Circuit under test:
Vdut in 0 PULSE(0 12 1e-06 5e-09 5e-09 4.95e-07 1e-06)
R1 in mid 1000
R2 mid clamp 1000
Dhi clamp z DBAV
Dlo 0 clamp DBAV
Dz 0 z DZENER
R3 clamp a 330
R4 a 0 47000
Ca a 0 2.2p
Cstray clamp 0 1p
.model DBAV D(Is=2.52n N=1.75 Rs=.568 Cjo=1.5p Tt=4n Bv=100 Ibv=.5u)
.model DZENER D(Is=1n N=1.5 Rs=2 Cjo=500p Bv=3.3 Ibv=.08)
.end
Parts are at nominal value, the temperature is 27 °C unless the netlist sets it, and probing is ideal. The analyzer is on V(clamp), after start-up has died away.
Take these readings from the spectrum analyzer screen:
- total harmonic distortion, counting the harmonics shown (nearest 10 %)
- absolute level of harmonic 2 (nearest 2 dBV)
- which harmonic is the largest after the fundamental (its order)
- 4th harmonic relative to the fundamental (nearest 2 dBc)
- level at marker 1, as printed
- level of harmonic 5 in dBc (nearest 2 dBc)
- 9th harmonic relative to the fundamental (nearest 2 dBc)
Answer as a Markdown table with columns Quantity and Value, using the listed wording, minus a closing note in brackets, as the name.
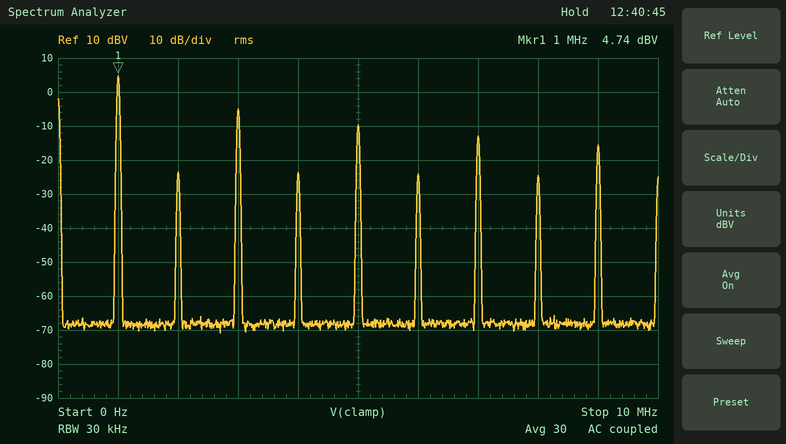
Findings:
| Quantity | Value |
|---|---|
| total harmonic distortion, counting the harmonics shown | 40 % |
| absolute level of harmonic 2 | -24 dBV |
| which harmonic is the largest after the fundamental | 3 |
| 4th harmonic relative to the fundamental | -28 dBc |
| level at marker 1, as printed | 4.74 dBV |
| level of harmonic 5 in dBc | -14 dBc |
| 9th harmonic relative to the fundamental | -20 dBc |
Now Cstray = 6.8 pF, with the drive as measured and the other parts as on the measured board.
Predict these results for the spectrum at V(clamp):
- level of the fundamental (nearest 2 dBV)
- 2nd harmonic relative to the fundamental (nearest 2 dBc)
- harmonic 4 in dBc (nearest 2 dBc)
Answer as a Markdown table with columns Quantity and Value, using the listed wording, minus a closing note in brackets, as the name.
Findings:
| Quantity | Value |
|---|---|
| level of the fundamental | 4 dBV |
| 2nd harmonic relative to the fundamental | -24 dBc |
| harmonic 4 in dBc | -24 dBc |
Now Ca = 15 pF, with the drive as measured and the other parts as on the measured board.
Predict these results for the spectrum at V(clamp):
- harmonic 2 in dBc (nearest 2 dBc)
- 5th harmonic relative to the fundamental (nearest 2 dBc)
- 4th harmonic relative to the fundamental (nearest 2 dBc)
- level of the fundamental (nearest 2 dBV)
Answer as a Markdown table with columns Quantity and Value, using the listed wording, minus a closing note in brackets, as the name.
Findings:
| Quantity | Value |
|---|---|
| harmonic 2 in dBc | -20 dBc |
| 5th harmonic relative to the fundamental | -16 dBc |
| 4th harmonic relative to the fundamental | -22 dBc |
| level of the fundamental | 4 dBV |
